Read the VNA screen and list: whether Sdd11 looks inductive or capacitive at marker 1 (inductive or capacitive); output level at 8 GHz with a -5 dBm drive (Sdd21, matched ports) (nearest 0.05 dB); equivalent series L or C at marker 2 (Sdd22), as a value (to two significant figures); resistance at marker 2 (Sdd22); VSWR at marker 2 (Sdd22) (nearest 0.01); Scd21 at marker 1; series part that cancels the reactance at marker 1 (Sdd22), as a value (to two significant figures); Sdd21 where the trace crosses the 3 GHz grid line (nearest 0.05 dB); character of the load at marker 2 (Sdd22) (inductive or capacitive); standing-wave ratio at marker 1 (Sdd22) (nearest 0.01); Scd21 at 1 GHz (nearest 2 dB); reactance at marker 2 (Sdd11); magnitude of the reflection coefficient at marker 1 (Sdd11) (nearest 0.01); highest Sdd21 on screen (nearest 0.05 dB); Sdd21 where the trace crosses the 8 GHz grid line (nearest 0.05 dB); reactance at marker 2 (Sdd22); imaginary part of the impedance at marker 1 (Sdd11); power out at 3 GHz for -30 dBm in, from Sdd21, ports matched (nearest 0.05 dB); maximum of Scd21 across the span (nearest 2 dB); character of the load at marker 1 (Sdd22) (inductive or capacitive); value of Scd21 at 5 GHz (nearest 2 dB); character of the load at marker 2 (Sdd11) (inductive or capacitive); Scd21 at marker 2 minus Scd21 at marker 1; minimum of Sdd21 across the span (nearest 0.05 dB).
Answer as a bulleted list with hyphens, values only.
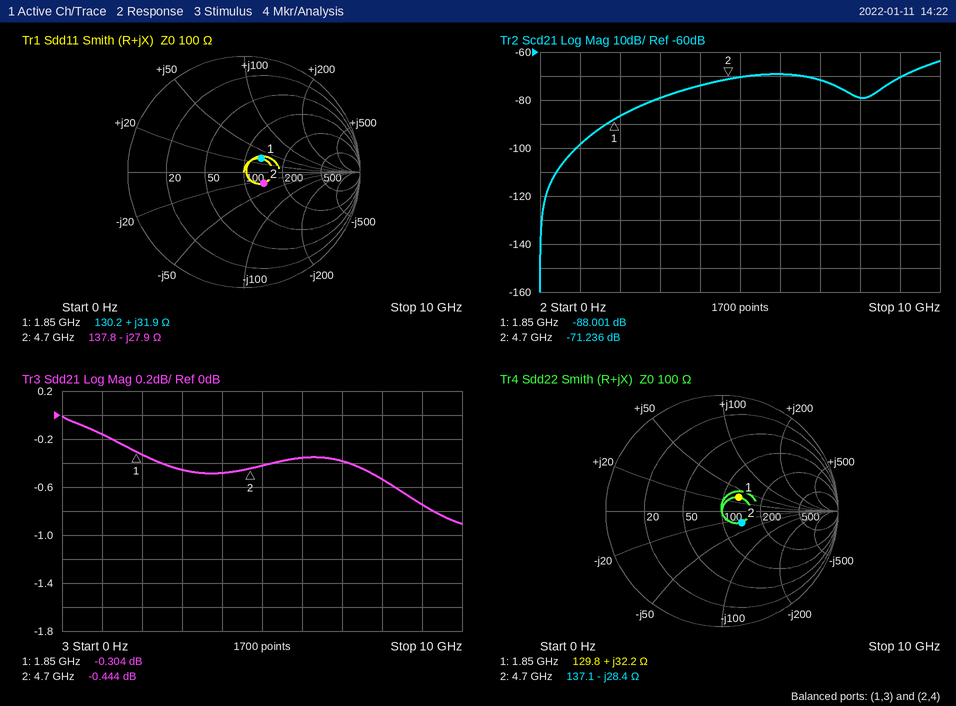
- inductive
- -5.55 dBm
- 1.2 pF
- 137.1 Ω
- 1.49
- -88.001 dB
- 2.7 pF
- -0.45 dB
- capacitive
- 1.47
- -98 dB
- -27.9 Ω
- 0.19
- 0.00 dB
- -0.55 dB
- -28.4 Ω
- +31.9 Ω
- -30.45 dBm
- -64 dB
- inductive
- -70 dB
- capacitive
- 16.765 dB
- -0.90 dB
